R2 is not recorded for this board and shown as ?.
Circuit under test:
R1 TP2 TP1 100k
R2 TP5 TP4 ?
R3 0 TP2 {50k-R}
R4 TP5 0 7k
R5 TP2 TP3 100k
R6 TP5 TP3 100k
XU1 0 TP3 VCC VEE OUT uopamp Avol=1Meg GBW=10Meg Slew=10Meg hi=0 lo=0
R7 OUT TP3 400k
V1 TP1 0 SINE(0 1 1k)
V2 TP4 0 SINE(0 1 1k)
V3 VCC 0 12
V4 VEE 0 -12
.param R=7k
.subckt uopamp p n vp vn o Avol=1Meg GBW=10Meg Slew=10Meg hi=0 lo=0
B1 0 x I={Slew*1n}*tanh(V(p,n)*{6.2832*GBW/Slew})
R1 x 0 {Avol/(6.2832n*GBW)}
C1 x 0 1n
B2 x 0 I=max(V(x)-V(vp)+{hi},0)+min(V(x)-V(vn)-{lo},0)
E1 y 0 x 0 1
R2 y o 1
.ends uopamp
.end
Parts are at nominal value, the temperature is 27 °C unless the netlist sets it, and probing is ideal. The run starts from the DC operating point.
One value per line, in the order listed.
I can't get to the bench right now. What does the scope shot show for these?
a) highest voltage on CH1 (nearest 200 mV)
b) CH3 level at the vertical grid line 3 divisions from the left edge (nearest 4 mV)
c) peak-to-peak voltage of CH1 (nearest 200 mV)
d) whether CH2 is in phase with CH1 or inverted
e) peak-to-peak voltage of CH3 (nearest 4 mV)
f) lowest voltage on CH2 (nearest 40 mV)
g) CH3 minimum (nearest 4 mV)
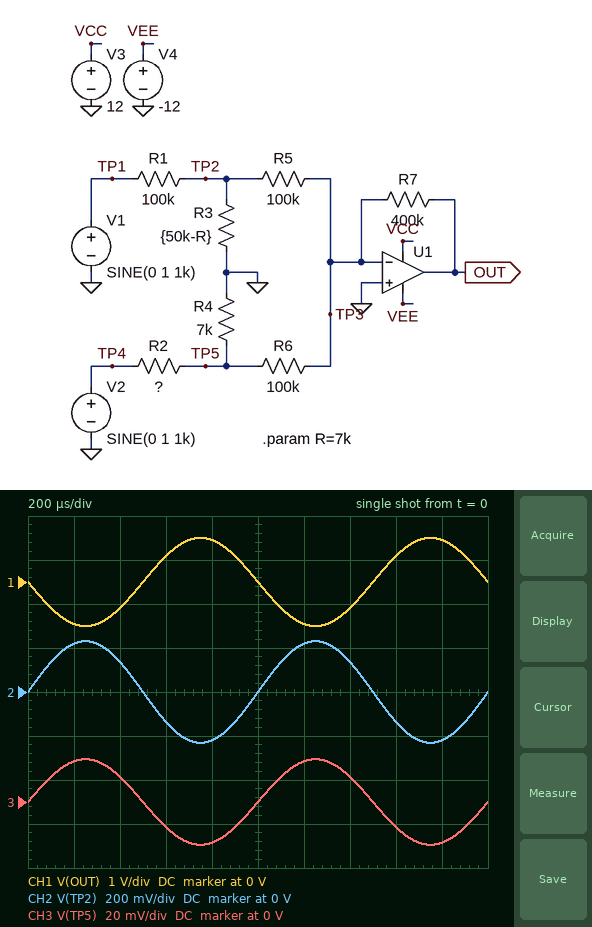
1.0 V
-12 mV
2.0 V
inverted
40 mV
-240 mV
-20 mV
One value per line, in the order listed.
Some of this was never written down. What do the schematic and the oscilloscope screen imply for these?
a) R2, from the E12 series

330 kΩ
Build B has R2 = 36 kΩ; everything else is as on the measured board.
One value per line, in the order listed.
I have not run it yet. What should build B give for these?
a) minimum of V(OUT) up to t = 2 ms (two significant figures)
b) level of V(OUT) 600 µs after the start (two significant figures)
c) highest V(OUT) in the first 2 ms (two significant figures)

-1.5 V
900 mV
1.5 V
